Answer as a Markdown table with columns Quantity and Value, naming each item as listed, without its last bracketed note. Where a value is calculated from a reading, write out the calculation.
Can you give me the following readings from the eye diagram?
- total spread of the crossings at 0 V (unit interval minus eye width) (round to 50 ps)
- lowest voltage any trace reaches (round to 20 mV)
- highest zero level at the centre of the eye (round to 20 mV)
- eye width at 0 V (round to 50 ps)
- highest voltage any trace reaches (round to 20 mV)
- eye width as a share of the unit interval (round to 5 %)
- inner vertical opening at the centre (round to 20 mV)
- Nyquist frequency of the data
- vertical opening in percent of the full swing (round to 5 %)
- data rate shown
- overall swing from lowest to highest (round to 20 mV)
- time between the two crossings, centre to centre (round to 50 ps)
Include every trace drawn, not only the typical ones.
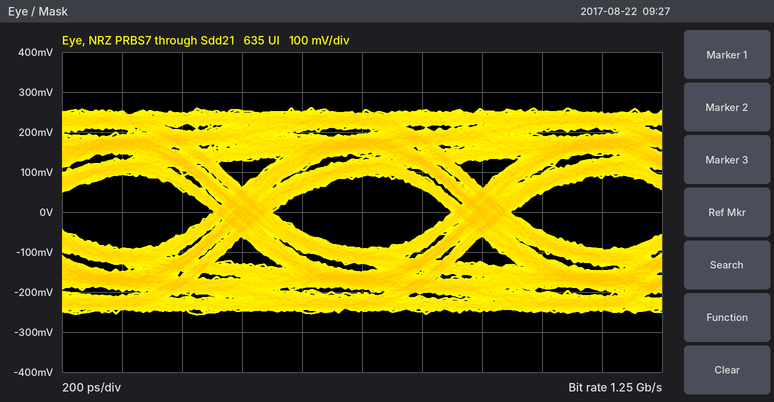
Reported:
| Quantity | Value |
|---|---|
| total spread of the crossings at 0 V (unit interval minus eye width) | 200 ps |
| lowest voltage any trace reaches | -260 mV |
| highest zero level at the centre of the eye | -100 mV |
| eye width at 0 V | 600 ps |
| highest voltage any trace reaches | 260 mV |
| eye width as a share of the unit interval | 600 ps / 800 ps ≈ 75 % |
| inner vertical opening at the centre | 180 mV |
| Nyquist frequency of the data | 625 MHz |
| vertical opening in percent of the full swing | 180 mV / 520 mV ≈ 35 % |
| data rate shown | 1.25 Gb/s |
| overall swing from lowest to highest | 520 mV |
| time between the two crossings, centre to centre | 800 ps |
